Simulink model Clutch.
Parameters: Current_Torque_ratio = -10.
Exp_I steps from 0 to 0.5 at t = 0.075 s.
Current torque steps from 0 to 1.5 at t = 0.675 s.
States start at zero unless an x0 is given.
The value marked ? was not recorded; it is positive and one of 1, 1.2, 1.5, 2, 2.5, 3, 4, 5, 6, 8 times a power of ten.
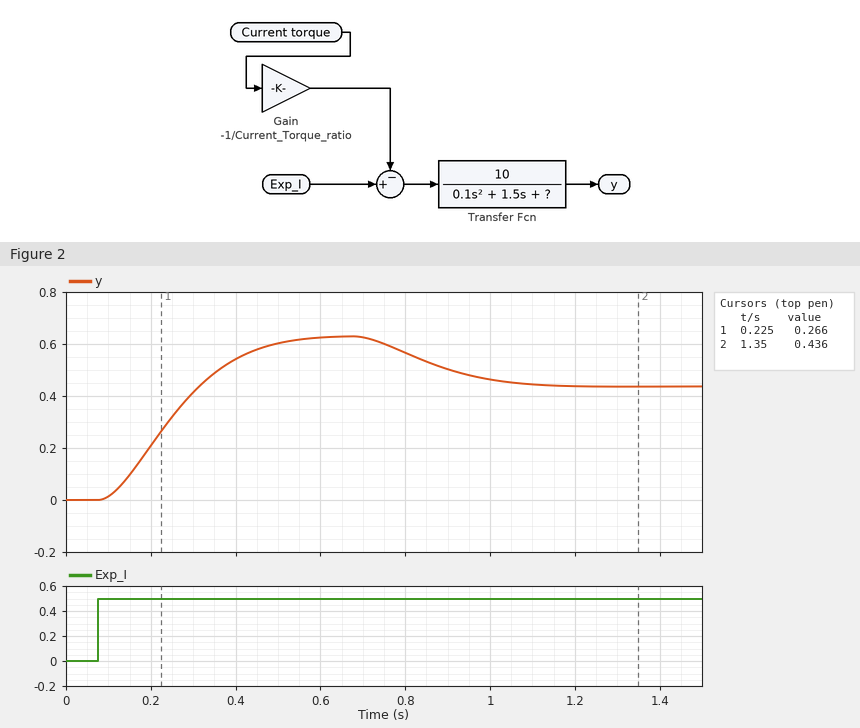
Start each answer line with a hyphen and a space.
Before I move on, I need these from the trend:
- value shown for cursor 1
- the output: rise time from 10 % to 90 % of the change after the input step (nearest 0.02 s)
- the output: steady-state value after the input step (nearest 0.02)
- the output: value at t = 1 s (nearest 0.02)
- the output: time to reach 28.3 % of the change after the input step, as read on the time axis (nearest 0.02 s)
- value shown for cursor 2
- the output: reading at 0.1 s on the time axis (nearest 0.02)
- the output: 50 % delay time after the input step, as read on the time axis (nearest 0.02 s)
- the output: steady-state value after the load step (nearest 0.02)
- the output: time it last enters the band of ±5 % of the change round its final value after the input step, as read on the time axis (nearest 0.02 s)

- 0.266
- 0.30 s
- 0.62
- 0.46
- 0.18 s
- 0.436
- 0.02
- 0.24 s
- 0.44
- 0.48 s
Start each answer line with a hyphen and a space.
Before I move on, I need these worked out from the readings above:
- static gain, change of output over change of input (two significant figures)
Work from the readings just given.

- 1.2
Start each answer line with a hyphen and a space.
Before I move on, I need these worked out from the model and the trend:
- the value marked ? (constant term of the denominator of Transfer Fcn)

- 8
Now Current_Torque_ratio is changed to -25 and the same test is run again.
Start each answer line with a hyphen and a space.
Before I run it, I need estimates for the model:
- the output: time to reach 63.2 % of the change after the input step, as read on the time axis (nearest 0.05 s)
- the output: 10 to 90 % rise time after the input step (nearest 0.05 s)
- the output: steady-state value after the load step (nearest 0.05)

- 0.30 s
- 0.30 s
- 0.55
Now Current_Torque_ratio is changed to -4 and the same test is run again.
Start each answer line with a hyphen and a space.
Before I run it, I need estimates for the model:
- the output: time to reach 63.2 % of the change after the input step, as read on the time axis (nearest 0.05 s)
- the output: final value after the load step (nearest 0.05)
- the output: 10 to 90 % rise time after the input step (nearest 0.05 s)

- 0.30 s
- 0.15
- 0.30 s
